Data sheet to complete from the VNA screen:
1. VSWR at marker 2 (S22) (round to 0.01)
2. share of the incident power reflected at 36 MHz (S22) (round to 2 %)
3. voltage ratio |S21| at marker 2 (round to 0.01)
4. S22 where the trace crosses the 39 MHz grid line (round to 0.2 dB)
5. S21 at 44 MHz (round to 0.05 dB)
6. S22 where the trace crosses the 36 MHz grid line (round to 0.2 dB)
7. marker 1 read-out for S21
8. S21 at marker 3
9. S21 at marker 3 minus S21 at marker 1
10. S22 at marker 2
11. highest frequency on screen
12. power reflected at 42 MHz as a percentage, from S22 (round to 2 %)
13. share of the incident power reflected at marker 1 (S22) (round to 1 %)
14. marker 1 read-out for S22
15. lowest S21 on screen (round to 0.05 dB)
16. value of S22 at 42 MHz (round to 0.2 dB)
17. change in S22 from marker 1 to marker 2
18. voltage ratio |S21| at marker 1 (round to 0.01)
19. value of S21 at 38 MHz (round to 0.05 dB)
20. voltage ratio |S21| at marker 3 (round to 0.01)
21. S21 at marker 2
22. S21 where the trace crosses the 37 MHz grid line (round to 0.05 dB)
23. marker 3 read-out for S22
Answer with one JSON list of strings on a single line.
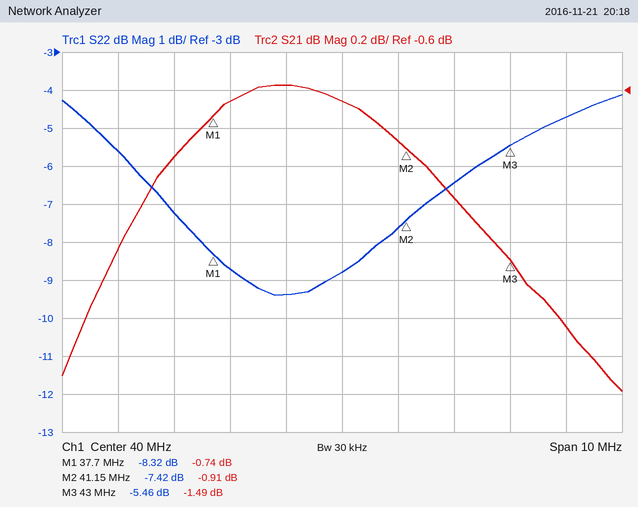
["2.48", "28 %", "0.90", "-9.4 dB", "-1.85 dB", "-5.6 dB", "-0.74 dB", "-1.49 dB", "-0.75 dB", "-7.42 dB", "45 MHz", "22 %", "15 %", "-8.32 dB", "-2.20 dB", "-6.4 dB", "0.90 dB", "0.92", "-0.65 dB", "0.84", "-0.91 dB", "-0.95 dB", "-5.46 dB"]
